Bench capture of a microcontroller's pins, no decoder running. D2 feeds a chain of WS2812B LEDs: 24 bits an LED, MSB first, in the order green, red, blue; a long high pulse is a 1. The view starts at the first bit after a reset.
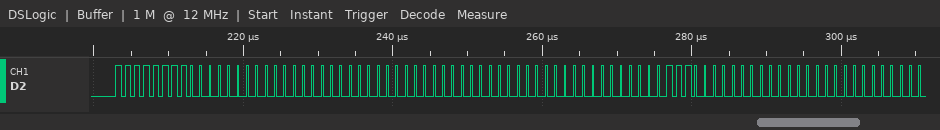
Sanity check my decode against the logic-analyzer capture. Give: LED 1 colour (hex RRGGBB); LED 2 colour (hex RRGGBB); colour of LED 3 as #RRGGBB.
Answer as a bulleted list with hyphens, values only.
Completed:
- #00FF00
- #000000
- #1C0000
